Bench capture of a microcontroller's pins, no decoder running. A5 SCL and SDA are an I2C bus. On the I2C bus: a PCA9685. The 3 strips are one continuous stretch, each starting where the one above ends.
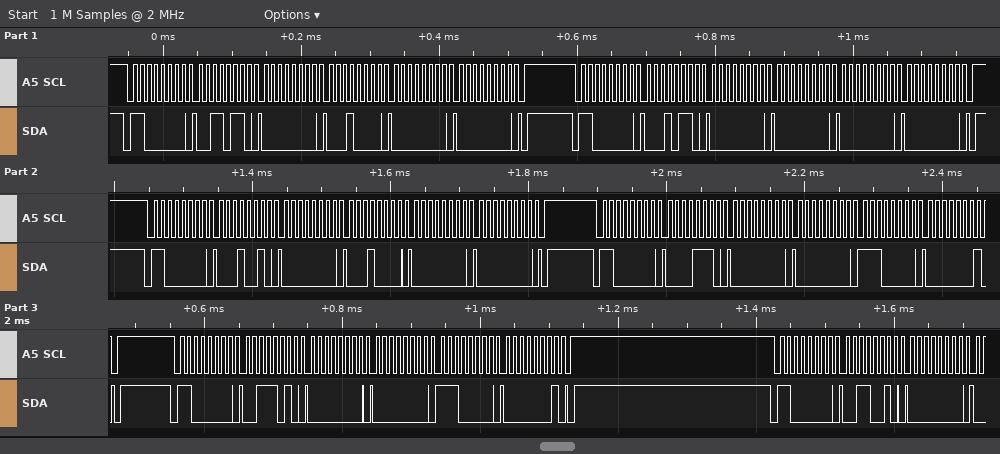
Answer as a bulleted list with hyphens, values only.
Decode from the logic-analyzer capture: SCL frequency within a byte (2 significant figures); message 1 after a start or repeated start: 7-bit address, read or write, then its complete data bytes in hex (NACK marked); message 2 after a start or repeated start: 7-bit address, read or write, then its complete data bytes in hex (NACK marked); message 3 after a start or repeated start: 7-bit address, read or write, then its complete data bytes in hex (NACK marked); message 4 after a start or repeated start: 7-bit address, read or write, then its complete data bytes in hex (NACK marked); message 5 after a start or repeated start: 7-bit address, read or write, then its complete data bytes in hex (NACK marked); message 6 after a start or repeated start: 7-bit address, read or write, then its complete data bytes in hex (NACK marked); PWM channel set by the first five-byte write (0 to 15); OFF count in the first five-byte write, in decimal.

- 100 kHz
- 0x60 write: 36 00 10 00 00
- 0x60 write: 16 00 00 00 00
- 0x60 write: 12 00 10 00 00
- 0x60 write: 0E 00 00 E0 01
- 0x60 write: 3A 00 00 E0 01
- 0x60 write: 32 00
- 12
- 0
